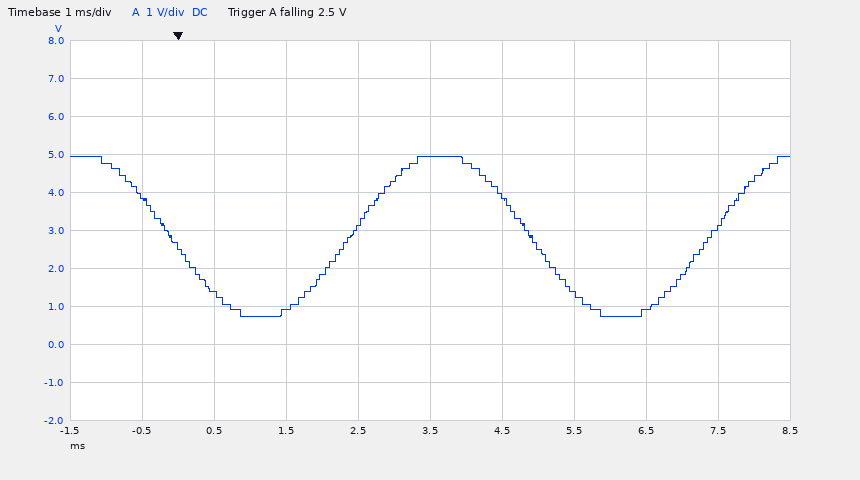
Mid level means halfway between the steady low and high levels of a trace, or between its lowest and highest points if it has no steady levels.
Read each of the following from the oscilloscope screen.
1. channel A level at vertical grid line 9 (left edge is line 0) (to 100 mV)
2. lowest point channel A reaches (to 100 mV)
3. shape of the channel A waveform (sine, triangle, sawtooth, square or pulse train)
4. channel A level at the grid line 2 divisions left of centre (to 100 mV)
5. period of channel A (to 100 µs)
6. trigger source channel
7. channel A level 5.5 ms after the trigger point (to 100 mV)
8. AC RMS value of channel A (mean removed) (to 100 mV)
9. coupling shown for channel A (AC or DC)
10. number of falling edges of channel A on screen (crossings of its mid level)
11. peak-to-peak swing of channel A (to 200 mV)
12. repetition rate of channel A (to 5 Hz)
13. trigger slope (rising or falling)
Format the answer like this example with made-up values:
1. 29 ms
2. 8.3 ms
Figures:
1. 3.1 V
2. 700 mV
3. sine
4. 900 mV
5. 5.0 ms
6. channel A
7. 1.3 V
8. 1.5 V
9. DC
10. 2
11. 4.2 V
12. 200 Hz
13. falling
